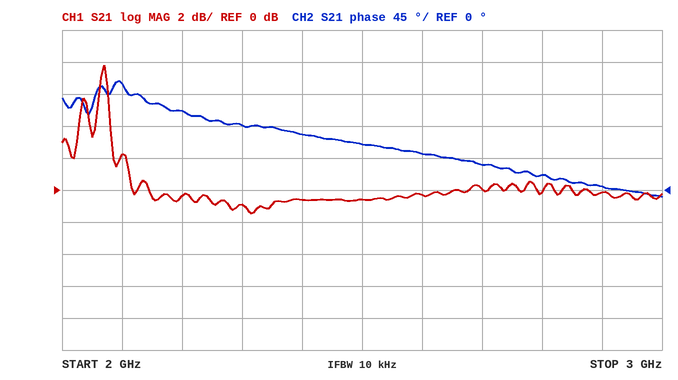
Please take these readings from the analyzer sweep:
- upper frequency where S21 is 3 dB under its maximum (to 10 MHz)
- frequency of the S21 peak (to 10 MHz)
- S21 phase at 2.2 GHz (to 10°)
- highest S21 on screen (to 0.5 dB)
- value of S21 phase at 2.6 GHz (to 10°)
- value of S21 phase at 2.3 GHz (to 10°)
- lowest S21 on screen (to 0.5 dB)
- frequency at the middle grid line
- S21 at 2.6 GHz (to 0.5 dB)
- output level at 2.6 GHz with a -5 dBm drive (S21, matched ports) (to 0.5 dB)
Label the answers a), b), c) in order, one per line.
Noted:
a) 2.08 GHz
b) 2.07 GHz
c) 110°
d) 8.0 dB
e) 50°
f) 90°
g) -1.5 dB
h) 2.5 GHz
i) -0.5 dB
j) -5.5 dBm
